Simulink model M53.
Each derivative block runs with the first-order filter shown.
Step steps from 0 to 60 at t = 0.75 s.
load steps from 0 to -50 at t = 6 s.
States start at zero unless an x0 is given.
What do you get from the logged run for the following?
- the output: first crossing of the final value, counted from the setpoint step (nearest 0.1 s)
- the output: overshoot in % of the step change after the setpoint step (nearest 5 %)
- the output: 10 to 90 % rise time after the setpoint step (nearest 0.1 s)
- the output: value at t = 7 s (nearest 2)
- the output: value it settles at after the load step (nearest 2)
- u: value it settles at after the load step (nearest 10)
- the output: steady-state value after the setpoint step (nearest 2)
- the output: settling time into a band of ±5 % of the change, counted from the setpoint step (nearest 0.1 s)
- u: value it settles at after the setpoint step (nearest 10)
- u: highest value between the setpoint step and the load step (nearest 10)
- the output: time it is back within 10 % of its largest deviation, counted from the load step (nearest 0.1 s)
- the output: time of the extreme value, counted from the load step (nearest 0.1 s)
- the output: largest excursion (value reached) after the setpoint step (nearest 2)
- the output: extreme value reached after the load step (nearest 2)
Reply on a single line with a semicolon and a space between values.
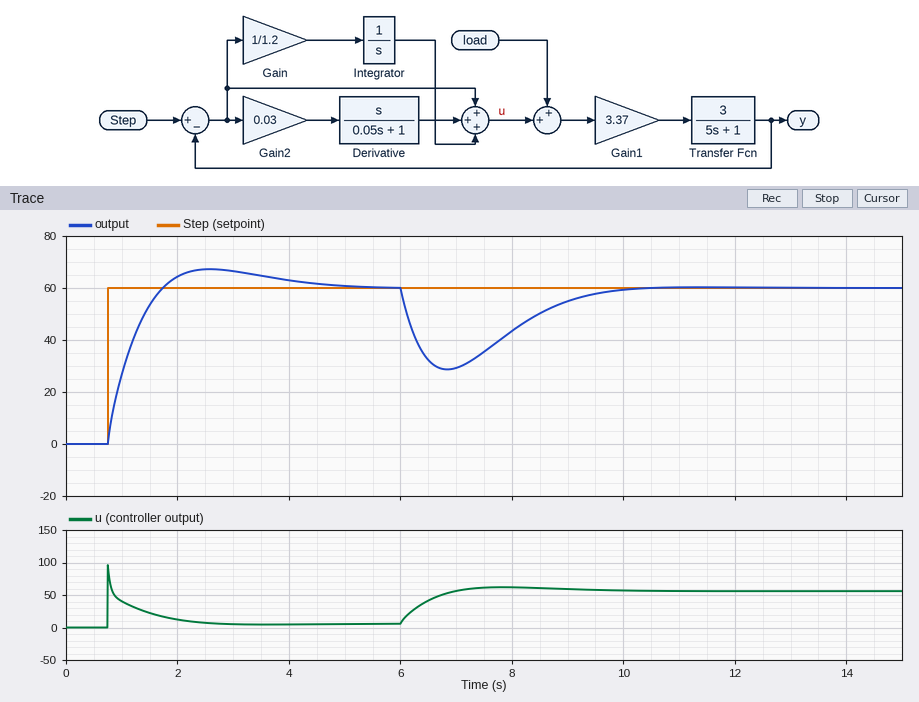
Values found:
1.0 s; 10 %; 0.7 s; 30; 60; 60; 60; 3.2 s; 10; 100; 3.3 s; 0.8 s; 68; 28
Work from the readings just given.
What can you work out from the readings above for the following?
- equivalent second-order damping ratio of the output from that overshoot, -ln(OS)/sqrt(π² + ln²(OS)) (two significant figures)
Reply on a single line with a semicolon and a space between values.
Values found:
0.59
